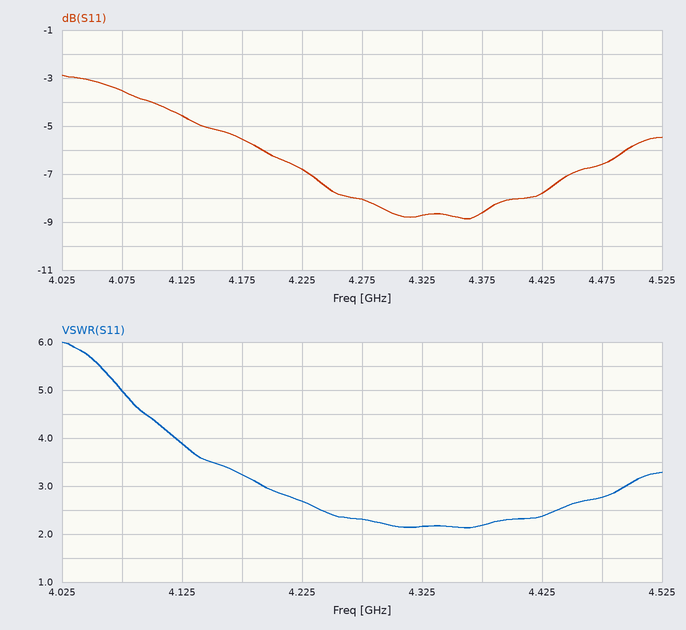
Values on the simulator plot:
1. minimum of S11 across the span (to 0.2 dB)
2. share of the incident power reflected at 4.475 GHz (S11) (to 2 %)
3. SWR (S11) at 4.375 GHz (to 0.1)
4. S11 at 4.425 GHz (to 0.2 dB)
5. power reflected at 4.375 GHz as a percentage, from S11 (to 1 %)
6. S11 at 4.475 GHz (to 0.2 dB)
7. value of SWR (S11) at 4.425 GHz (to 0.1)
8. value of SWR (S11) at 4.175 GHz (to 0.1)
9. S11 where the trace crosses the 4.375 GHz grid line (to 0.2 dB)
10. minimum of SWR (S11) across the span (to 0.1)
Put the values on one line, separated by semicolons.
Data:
-8.8 dB; 22 %; 2.2; -7.8 dB; 14 %; -6.6 dB; 2.4; 3.2; -8.6 dB; 2.1
